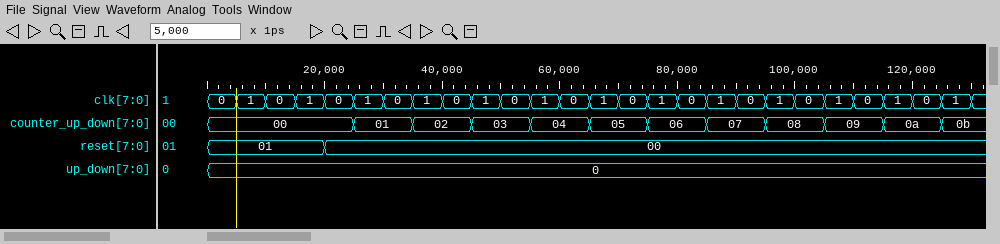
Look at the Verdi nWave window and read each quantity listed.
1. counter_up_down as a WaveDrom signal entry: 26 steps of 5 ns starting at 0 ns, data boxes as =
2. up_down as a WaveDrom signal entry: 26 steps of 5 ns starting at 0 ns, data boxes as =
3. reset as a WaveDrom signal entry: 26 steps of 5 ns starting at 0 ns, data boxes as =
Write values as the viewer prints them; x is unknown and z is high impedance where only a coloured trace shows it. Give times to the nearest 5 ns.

{name: 'counter_up_down', wave: '=....=.=.=.=.=.=.=.=.=.=.=', data: '00 01 02 03 04 05 06 07 08 09 0a 0b'}
{name: 'up_down', wave: '=.........................', data: '0'}
{name: 'reset', wave: '=...=.....................', data: '01 00'}
